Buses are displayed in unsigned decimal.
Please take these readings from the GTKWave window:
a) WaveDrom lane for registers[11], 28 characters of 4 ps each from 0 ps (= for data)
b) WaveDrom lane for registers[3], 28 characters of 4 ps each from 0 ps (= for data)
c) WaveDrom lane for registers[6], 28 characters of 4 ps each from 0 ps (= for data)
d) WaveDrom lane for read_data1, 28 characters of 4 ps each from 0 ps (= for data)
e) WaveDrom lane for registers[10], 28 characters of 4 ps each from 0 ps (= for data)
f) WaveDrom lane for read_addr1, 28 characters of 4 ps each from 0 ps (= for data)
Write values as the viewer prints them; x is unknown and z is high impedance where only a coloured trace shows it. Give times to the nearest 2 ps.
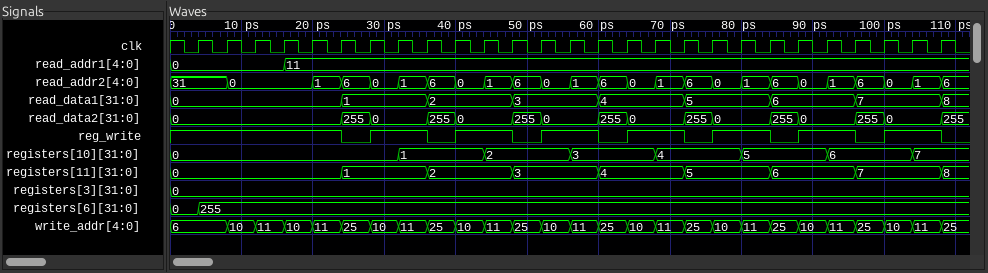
{name: 'registers[11]', wave: '=.....=..=..=..=..=..=..=..=', data: '0 1 2 3 4 5 6 7 8'}
{name: 'registers[3]', wave: '=...........................', data: '0'}
{name: 'registers[6]', wave: '==..........................', data: '0 255'}
{name: 'read_data1', wave: '=.....=..=..=..=..=..=..=..=', data: '0 1 2 3 4 5 6 7 8'}
{name: 'registers[10]', wave: '=.......=..=..=..=..=..=..=.', data: '0 1 2 3 4 5 6 7'}
{name: 'read_addr1', wave: '=...=.......................', data: '0 11'}
